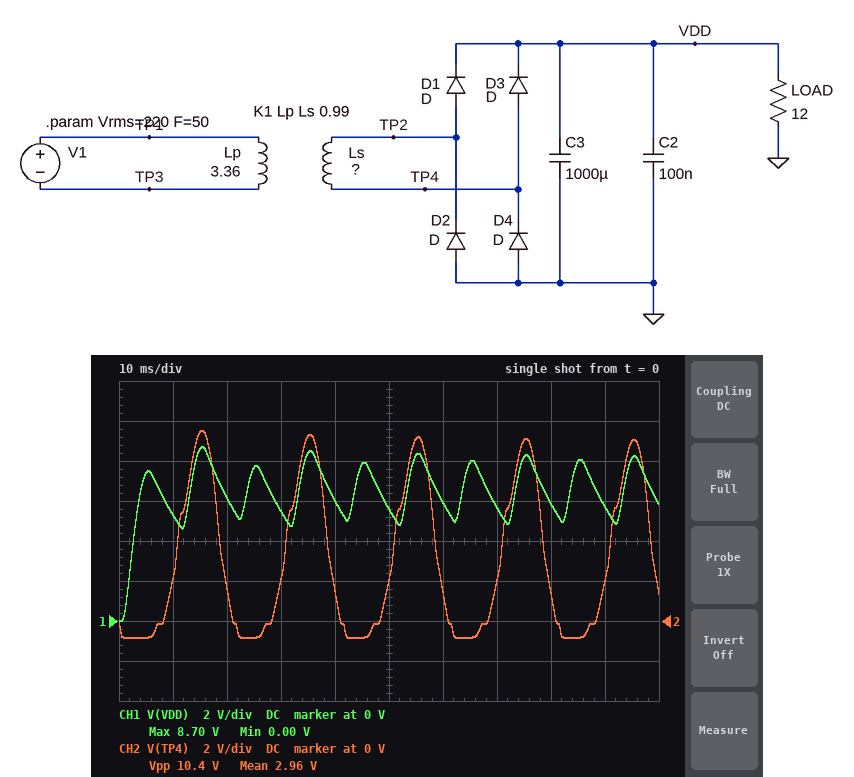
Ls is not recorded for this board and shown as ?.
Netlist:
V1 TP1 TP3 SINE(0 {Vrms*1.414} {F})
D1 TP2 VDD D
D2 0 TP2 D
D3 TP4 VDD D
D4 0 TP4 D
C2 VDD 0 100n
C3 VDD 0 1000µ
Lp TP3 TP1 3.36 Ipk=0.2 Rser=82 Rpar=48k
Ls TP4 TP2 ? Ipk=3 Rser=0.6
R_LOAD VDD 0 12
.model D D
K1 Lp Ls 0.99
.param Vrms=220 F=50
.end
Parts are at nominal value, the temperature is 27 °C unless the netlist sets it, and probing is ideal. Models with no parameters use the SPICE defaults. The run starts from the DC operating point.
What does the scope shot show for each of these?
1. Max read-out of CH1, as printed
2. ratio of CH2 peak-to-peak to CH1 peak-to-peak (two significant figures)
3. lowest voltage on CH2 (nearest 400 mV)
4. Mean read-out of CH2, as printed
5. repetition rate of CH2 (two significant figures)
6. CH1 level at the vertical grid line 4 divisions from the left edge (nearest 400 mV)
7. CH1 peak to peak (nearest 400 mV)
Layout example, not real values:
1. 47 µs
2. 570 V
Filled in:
1. 8.70 V
2. 1.2
3. -800 mV
4. 2.96 V
5. 50 Hz
6. 6.0 V
7. 8.8 V
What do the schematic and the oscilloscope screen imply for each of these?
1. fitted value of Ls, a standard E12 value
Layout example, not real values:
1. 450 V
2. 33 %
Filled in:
1. 3.9 mH
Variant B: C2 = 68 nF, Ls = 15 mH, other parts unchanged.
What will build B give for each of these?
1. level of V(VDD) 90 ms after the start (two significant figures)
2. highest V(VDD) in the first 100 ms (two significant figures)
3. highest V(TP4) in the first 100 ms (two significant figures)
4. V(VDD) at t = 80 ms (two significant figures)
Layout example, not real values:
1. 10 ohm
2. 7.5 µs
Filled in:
1. 12 V
2. 18 V
3. 19 V
4. 13 V
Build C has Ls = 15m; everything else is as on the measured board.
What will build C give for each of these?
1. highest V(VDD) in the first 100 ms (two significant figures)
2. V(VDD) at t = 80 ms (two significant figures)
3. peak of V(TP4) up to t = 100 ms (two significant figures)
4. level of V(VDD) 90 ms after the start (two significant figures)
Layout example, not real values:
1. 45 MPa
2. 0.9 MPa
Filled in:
1. 18 V
2. 13 V
3. 19 V
4. 12 V
